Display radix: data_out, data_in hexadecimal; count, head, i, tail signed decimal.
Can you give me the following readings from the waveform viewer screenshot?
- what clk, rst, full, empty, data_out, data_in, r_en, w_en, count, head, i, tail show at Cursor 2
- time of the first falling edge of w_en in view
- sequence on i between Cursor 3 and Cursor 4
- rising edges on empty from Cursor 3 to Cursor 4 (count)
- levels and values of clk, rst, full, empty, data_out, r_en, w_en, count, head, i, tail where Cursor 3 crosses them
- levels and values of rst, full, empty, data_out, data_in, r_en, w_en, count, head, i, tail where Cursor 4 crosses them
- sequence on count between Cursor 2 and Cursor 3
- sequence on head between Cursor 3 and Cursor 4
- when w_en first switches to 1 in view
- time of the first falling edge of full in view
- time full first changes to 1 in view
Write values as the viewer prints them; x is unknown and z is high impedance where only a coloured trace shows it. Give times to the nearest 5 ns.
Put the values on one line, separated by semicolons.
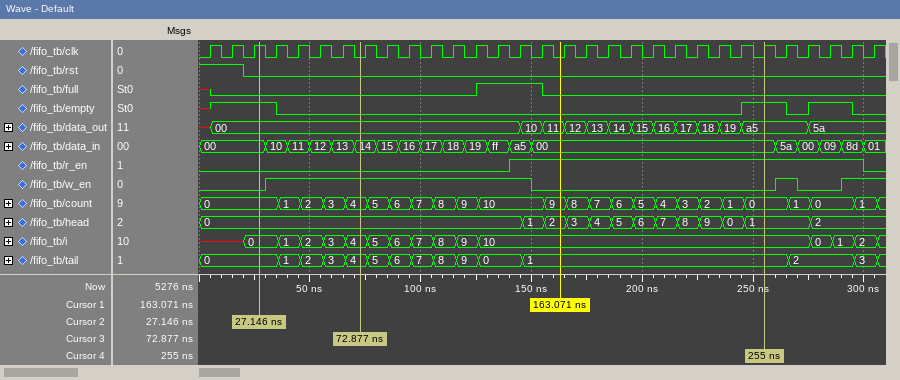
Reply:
clk=1, rst=0, full=0, empty=1, data_out=00, data_in=00, r_en=0, w_en=0, count=0, head=0, i=0, tail=0; 150 ns; 4, 5, 6, 7, 8, 9, 10; 1; clk=0, rst=0, full=0, empty=0, data_out=00, r_en=0, w_en=1, count=4, head=0, i=4, tail=4; rst=0, full=0, empty=1, data_out=a5, data_in=00, r_en=1, w_en=0, count=0, head=1, i=10, tail=1; 0, 1, 2, 3, 4; 0, 1, 2, 3, 4, 5, 6, 7, 8, 9, 0, 1; 30 ns; 155 ns; 125 ns
